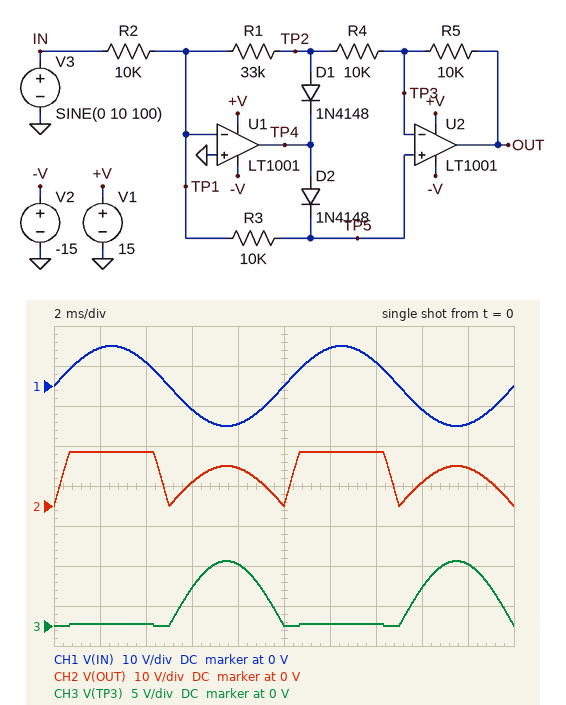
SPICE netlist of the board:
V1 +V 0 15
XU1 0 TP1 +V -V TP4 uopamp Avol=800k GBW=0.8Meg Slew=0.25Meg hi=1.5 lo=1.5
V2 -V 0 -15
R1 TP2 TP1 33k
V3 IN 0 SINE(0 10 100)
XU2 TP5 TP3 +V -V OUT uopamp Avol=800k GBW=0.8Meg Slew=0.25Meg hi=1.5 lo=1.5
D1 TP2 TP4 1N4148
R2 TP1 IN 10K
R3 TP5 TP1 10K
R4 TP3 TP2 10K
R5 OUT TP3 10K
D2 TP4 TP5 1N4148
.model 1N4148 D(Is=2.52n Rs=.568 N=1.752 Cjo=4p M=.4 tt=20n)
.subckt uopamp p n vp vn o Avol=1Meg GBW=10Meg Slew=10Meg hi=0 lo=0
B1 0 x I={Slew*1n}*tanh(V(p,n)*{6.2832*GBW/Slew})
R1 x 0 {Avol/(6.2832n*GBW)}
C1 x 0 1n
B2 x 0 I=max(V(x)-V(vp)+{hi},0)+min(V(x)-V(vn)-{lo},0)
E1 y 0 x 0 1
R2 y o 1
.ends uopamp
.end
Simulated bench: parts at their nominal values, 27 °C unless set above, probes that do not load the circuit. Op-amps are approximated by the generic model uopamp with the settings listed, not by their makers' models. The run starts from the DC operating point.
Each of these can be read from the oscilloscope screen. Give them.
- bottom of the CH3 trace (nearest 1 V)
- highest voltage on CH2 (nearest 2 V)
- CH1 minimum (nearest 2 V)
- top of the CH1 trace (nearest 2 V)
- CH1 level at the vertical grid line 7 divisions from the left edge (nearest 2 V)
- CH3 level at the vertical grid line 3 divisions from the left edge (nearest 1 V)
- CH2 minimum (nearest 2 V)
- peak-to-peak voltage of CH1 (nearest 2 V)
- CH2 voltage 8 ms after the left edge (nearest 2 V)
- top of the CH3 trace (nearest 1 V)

0 V
14 V
-10 V
10 V
6 V
5 V
0 V
20 V
10 V
8 V
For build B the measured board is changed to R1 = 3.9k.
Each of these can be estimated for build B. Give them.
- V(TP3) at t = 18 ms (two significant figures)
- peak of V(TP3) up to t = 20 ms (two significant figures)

5.5 V
5.8 V
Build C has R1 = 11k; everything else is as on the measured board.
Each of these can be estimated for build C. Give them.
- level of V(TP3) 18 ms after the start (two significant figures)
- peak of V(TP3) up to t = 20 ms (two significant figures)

6.4 V
6.8 V
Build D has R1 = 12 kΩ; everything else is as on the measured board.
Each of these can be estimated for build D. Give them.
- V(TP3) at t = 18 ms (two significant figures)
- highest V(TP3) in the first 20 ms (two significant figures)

6.5 V
6.9 V
